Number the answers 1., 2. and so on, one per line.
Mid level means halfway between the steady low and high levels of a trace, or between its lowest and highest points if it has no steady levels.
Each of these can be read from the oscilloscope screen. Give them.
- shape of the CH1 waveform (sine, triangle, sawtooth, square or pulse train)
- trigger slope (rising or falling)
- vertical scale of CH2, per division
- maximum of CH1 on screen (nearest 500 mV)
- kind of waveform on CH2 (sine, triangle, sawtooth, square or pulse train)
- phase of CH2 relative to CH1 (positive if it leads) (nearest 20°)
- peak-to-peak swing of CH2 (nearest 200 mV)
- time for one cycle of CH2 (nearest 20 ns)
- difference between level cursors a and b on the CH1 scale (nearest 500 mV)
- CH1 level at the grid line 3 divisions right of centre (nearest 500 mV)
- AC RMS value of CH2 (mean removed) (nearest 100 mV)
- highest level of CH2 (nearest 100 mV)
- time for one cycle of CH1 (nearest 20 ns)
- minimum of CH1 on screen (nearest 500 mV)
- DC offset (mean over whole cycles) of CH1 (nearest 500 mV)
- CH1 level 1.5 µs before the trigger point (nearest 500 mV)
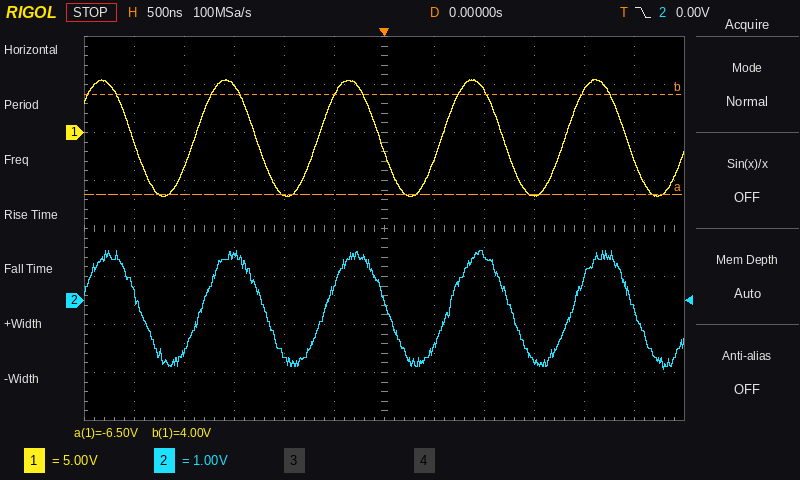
1. sine
2. falling
3. 1 V
4. 5.5 V
5. sine
6. -20°
7. 2.4 V
8. 1.24 µs
9. 10.5 V
10. -6.5 V
11. 800 mV
12. 1.0 V
13. 1.24 µs
14. -6.5 V
15. -500 mV
16. 5.0 V
